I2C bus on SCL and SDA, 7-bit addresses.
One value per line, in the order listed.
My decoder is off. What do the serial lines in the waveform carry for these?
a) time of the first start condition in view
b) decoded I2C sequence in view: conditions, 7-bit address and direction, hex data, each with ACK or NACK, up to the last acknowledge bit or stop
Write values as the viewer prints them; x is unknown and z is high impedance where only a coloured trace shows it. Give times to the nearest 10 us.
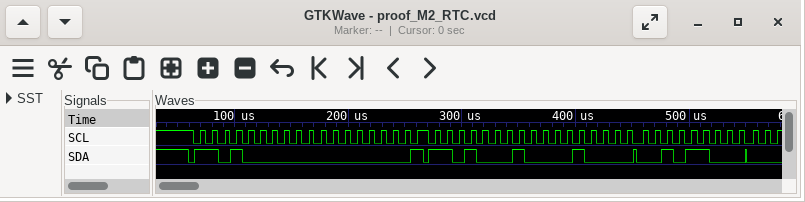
60 us
start, address 68 write ACK, 00 ACK, repeated start, address 68 read ACK, 10 ACK, 58 ACK
